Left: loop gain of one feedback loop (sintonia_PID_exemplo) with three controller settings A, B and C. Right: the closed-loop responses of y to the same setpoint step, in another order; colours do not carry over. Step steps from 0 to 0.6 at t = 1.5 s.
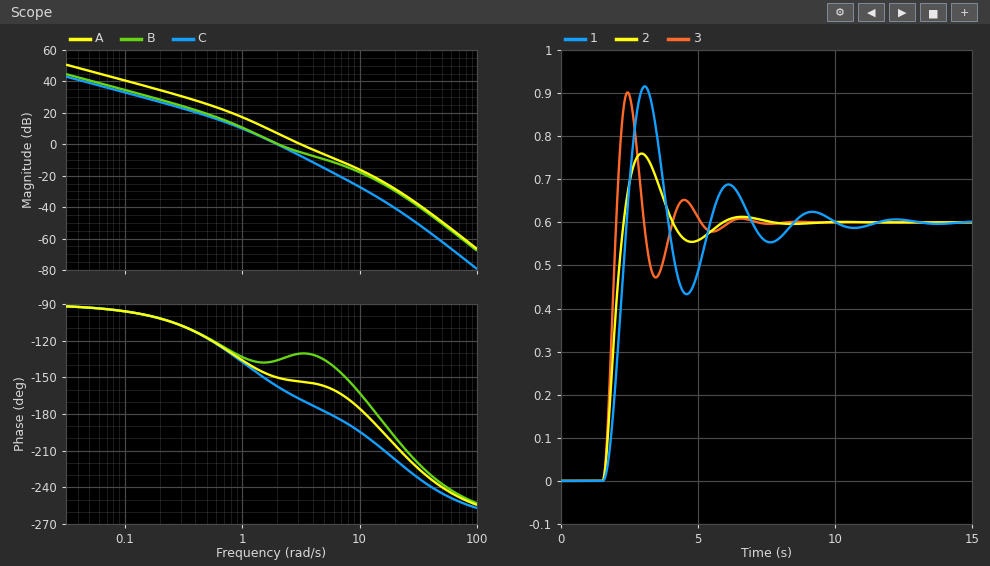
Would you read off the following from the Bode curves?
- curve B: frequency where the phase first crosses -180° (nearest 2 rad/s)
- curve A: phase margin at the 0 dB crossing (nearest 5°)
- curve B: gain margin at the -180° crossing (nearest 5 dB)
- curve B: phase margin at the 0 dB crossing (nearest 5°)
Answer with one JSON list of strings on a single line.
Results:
["14 rad/s", "25°", "25 dB", "45°"]
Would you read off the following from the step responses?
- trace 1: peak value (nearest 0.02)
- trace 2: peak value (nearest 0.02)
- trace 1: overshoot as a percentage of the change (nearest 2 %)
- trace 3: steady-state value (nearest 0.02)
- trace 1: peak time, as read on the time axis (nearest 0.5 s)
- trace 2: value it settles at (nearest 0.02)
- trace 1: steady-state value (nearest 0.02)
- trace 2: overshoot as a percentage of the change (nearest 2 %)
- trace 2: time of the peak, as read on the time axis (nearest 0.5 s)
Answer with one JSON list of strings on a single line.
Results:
["0.92", "0.76", "52 %", "0.60", "3.0 s", "0.60", "0.60", "26 %", "3.0 s"]
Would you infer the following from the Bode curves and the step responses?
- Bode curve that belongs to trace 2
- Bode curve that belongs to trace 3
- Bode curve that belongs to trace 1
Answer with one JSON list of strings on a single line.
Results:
["B", "A", "C"]
